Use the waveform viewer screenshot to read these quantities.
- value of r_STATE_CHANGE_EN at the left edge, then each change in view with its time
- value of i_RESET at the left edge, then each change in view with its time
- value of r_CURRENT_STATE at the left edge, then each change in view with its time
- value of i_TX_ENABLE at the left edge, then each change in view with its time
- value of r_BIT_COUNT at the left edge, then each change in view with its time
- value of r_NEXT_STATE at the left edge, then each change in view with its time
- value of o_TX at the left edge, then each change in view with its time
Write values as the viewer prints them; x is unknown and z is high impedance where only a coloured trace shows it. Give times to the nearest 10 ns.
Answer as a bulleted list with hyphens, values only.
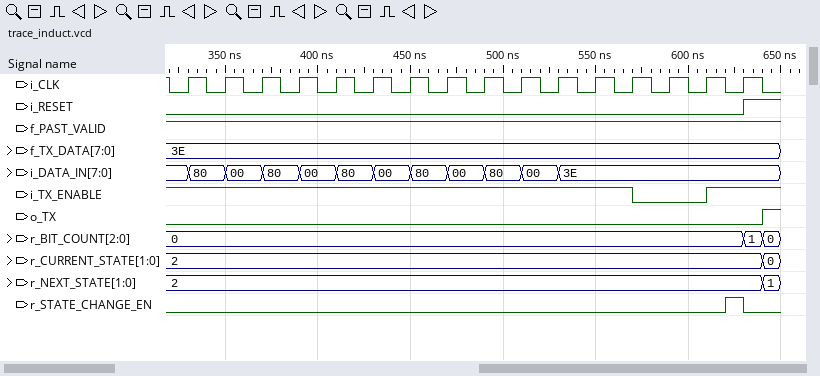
- 0, 1 at 620 ns, 0 at 630 ns
- 0, 1 at 630 ns
- 2, 0 at 640 ns
- 1, 0 at 570 ns, 1 at 610 ns
- 0, 1 at 630 ns, 0 at 640 ns
- 2, 1 at 640 ns
- 0, 1 at 640 ns
